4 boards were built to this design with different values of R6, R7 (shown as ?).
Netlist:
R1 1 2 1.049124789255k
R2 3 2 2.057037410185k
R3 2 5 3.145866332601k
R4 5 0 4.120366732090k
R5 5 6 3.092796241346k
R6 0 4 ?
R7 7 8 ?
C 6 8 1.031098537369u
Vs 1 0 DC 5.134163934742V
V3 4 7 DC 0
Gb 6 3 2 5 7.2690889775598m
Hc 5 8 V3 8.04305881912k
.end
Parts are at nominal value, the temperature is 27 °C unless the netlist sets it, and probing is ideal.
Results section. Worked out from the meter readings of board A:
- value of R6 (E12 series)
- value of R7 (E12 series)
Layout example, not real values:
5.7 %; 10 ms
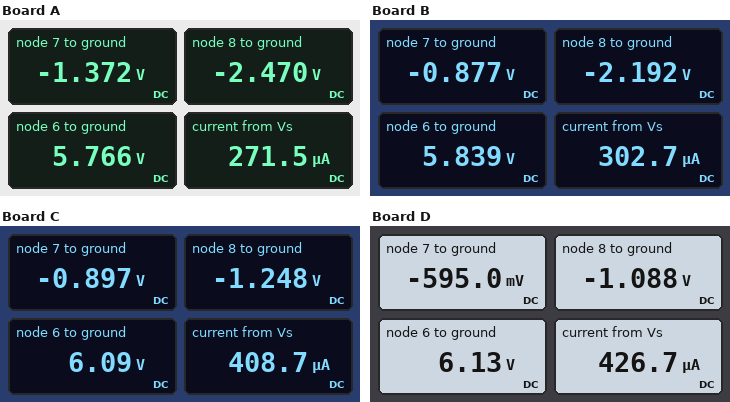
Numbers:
1.5 kΩ; 1.2 kΩ
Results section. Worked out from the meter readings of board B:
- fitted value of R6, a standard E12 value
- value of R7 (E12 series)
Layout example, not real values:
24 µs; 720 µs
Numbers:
1 kΩ; 1.5 kΩ
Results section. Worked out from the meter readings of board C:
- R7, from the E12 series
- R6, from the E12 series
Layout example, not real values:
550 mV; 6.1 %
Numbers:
470 Ω; 1.2 kΩ
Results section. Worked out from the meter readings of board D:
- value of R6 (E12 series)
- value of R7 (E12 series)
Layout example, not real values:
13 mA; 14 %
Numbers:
820 Ω; 680 Ω
